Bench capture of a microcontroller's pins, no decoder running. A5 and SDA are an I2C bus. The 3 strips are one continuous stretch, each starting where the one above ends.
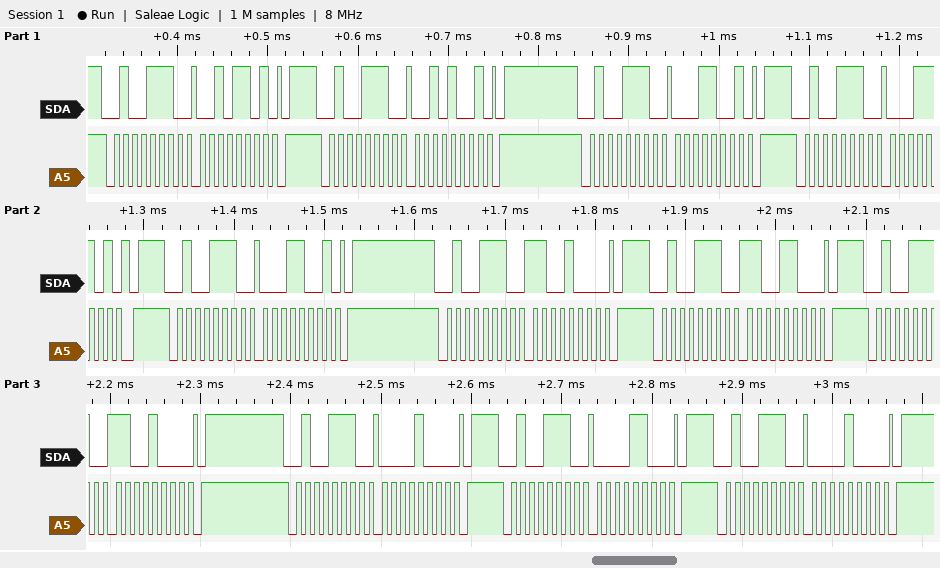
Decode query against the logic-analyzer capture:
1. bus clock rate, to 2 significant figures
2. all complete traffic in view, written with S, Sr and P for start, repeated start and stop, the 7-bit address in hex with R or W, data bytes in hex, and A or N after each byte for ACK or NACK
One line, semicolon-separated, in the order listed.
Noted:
100 kHz; S 27W A 2D A P S 27W A 29 A P S 27W A 19 A P S 27W A 1D A P S 27W A 19 A P S 27W A C8 A P S 27W A CC A P S 27W A C8 A P S 27W A 08 A P S 27W A 0C A P S 27W A 08 A P
